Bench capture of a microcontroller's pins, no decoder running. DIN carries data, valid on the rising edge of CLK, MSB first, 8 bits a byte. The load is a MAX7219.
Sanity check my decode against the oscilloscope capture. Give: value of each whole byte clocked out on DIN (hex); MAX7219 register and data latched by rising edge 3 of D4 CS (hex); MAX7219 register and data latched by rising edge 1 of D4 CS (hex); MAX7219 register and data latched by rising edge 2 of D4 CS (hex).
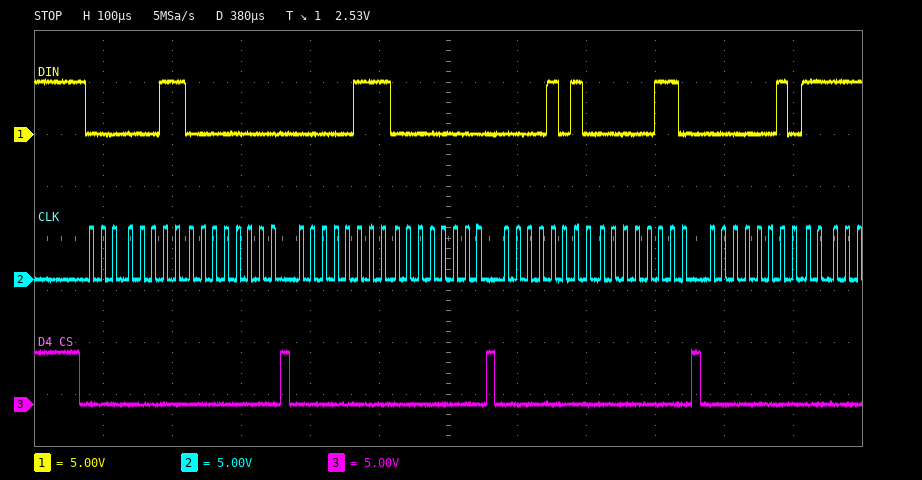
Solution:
03 00 07 00 0A 06 02
register 0xA, data 0x06
register 0x3, data 0x00
register 0x7, data 0x00
